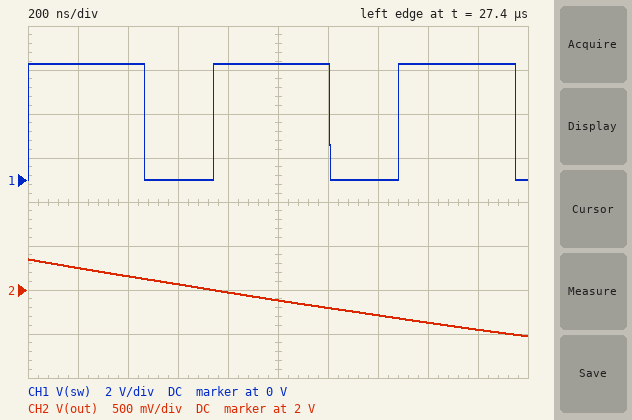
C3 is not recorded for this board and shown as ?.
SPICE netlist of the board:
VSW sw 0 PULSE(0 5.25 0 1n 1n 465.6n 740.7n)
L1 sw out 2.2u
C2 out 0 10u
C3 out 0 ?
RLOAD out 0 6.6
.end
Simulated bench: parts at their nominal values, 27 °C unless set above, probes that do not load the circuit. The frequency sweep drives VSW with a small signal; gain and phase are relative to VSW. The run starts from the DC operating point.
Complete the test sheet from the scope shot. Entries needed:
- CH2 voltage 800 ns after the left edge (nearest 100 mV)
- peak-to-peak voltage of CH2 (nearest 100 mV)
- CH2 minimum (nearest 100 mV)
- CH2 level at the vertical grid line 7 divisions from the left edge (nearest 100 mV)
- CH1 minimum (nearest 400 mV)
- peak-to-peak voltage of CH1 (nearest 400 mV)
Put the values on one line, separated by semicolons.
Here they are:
2.0 V; 900 mV; 1.5 V; 1.7 V; 0 V; 5.2 V
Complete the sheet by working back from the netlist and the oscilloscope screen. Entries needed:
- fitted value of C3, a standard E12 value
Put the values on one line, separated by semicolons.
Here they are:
3.3 µF
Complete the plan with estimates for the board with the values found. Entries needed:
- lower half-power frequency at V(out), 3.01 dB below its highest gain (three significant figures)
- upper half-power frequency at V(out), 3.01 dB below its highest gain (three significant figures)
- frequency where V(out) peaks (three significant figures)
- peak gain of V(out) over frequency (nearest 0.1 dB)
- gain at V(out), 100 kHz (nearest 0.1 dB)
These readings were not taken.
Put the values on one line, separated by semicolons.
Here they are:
28.5 kHz; 30.3 kHz; 29.4 kHz; 24.2 dB; -20.5 dB
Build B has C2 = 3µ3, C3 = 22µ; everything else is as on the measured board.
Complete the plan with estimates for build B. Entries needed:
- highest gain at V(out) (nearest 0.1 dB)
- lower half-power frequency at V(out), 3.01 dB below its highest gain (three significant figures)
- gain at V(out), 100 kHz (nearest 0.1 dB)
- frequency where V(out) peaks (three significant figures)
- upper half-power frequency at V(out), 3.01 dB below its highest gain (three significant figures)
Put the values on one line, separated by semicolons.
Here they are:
27.0 dB; 20.8 kHz; -26.4 dB; 21.3 kHz; 21.8 kHz
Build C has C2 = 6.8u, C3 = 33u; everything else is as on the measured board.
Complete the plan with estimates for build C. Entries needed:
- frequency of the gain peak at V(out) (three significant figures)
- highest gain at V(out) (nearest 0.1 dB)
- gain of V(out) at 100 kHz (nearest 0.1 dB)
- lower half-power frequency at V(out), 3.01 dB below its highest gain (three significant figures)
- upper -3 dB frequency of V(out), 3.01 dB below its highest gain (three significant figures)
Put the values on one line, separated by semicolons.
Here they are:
17.0 kHz; 29.0 dB; -30.5 dB; 16.7 kHz; 17.3 kHz
